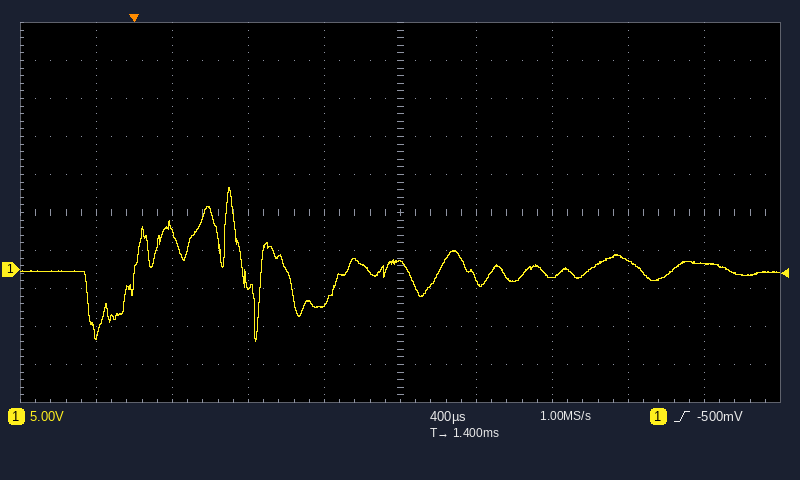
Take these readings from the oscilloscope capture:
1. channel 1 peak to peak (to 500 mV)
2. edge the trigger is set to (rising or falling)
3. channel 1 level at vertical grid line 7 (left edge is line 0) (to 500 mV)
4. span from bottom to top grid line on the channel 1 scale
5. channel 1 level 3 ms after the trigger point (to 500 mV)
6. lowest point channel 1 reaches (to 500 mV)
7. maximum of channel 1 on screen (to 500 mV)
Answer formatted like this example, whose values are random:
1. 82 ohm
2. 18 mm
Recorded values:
1. 20.5 V
2. rising
3. -1.0 V
4. 50 V
5. 1.0 V
6. -9.5 V
7. 11.0 V
